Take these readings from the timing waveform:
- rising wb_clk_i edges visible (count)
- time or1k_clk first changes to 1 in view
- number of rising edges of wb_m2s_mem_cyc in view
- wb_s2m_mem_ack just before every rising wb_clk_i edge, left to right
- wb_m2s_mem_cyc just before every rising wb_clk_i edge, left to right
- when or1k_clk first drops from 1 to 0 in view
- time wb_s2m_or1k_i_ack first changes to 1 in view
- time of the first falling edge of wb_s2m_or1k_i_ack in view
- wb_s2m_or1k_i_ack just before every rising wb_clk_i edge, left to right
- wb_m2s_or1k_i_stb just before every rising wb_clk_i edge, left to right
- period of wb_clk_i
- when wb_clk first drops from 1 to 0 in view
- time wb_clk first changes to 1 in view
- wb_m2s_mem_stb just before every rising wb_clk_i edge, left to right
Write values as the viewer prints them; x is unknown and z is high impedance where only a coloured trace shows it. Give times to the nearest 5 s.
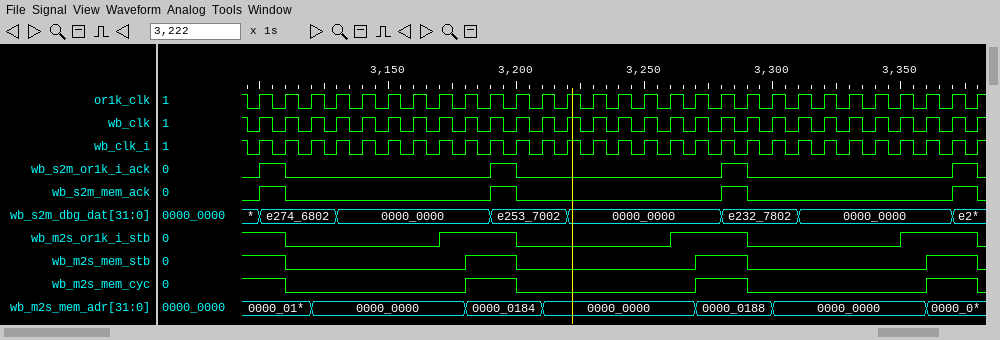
29
3100 s
3
0 1 0 0 0 0 0 0 0 0 1 0 0 0 0 0 0 0 0 1 0 0 0 0 0 0 0 0 1
1 1 0 0 0 0 0 0 0 1 1 0 0 0 0 0 0 0 1 1 0 0 0 0 0 0 0 1 1
3095 s
3100 s
3110 s
0 1 0 0 0 0 0 0 0 0 1 0 0 0 0 0 0 0 0 1 0 0 0 0 0 0 0 0 1
1 1 0 0 0 0 0 0 1 1 1 0 0 0 0 0 0 1 1 1 0 0 0 0 0 0 1 1 1
10 s
3095 s
3100 s
1 1 0 0 0 0 0 0 0 1 1 0 0 0 0 0 0 0 1 1 0 0 0 0 0 0 0 1 1
